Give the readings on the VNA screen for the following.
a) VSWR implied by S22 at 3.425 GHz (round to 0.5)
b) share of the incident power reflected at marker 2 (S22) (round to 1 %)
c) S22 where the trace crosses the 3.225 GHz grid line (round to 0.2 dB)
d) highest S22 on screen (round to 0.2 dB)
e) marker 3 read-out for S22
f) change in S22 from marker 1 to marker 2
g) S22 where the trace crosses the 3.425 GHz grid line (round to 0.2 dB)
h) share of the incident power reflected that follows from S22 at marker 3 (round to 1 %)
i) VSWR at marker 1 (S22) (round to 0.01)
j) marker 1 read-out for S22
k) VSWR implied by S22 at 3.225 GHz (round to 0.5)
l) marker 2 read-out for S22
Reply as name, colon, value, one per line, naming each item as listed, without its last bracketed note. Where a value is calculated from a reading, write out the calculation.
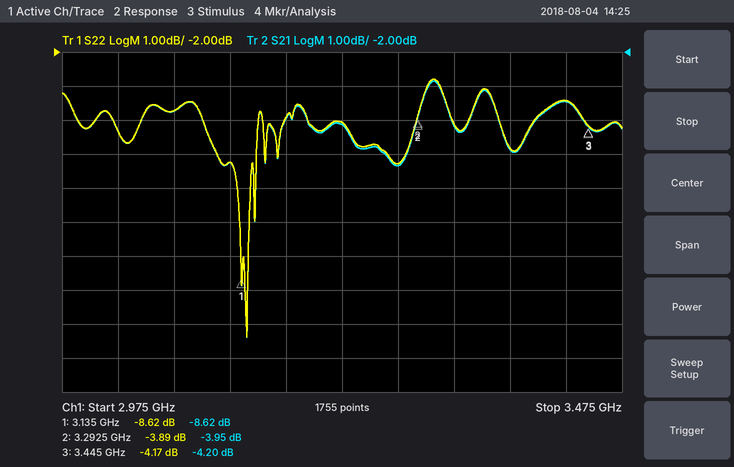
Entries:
VSWR implied by S22 at 3.425 GHz: |Γ| = 10^(-3.4/20) = 0.6761; VSWR = (1 + 0.6761)/(1 − 0.6761) ≈ 5.17, so 5.0 to the nearest 0.5
share of the incident power reflected at marker 2 (S22): 10^(-3.89/10) ≈ 41 %
S22 where the trace crosses the 3.225 GHz grid line: -4.0 dB
highest S22 on screen: -2.8 dB
marker 3 read-out for S22: -4.17 dB
change in S22 from marker 1 to marker 2: -3.89 − (-8.62) = 4.73 dB
S22 where the trace crosses the 3.425 GHz grid line: -3.4 dB
share of the incident power reflected that follows from S22 at marker 3: 10^(-4.17/10) ≈ 38 %
VSWR at marker 1 (S22): (1 + 0.3707)/(1 − 0.3707) ≈ 2.18
marker 1 read-out for S22: -8.62 dB
VSWR implied by S22 at 3.225 GHz: |Γ| = 10^(-4/20) = 0.6310; VSWR = (1 + 0.6310)/(1 − 0.6310) ≈ 4.42, so 4.5 to the nearest 0.5
marker 2 read-out for S22: -3.89 dB
